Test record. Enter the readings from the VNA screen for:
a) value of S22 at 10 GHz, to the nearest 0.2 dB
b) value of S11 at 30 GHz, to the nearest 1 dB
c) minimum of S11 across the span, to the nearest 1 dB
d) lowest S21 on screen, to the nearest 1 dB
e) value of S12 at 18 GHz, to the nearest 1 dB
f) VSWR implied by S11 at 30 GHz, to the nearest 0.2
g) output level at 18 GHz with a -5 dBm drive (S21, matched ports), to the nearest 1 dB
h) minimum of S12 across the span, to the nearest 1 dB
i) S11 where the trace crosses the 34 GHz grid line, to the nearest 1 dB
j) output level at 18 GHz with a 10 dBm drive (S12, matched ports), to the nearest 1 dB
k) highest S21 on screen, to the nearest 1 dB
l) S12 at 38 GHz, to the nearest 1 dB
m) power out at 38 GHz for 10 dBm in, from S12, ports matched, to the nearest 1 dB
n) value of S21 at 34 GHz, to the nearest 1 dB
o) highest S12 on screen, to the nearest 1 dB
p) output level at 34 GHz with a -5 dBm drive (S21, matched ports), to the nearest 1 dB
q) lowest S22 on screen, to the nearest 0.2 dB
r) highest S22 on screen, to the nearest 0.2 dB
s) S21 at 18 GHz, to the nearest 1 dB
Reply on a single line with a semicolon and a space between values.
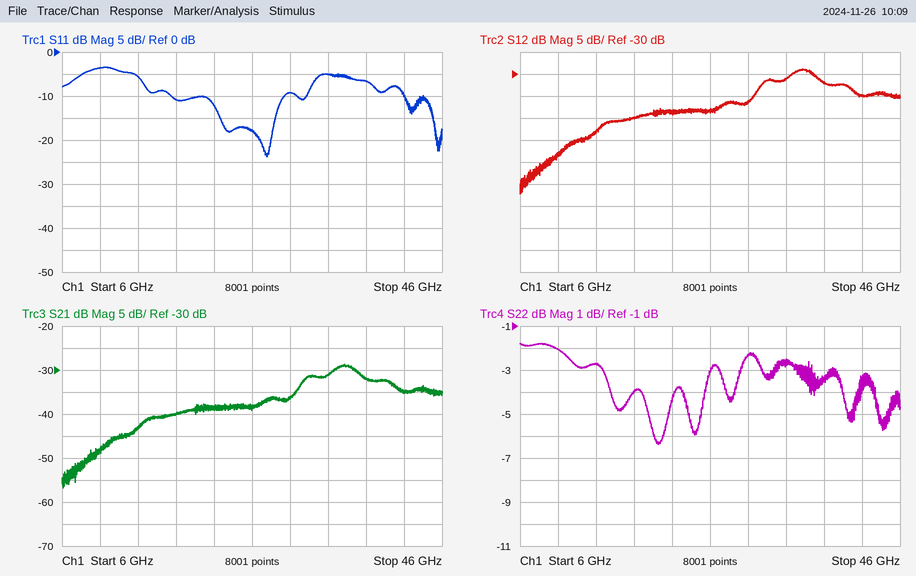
-2.0 dB; -9 dB; -24 dB; -57 dB; -40 dB; 2.0; -45 dBm; -57 dB; -5 dB; -30 dBm; -29 dB; -32 dB; -22 dBm; -31 dB; -29 dB; -36 dBm; -6.4 dB; -1.8 dB; -40 dB
